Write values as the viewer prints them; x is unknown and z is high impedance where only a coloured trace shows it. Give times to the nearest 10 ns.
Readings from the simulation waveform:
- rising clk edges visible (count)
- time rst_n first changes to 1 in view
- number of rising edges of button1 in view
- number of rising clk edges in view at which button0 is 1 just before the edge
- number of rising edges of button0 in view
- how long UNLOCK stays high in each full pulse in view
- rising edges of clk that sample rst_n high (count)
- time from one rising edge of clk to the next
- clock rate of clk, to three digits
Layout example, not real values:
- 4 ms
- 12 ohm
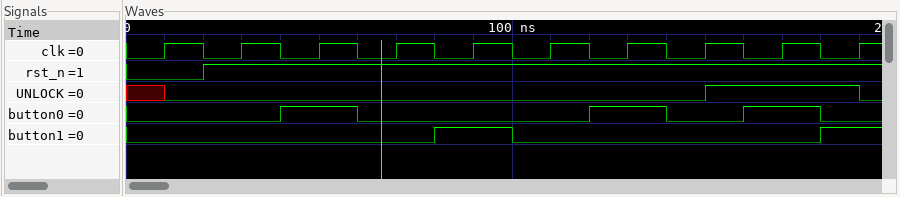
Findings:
- 10
- 20 ns
- 2
- 3
- 3
- 40 ns
- 9
- 20 ns
- 50.0 MHz
